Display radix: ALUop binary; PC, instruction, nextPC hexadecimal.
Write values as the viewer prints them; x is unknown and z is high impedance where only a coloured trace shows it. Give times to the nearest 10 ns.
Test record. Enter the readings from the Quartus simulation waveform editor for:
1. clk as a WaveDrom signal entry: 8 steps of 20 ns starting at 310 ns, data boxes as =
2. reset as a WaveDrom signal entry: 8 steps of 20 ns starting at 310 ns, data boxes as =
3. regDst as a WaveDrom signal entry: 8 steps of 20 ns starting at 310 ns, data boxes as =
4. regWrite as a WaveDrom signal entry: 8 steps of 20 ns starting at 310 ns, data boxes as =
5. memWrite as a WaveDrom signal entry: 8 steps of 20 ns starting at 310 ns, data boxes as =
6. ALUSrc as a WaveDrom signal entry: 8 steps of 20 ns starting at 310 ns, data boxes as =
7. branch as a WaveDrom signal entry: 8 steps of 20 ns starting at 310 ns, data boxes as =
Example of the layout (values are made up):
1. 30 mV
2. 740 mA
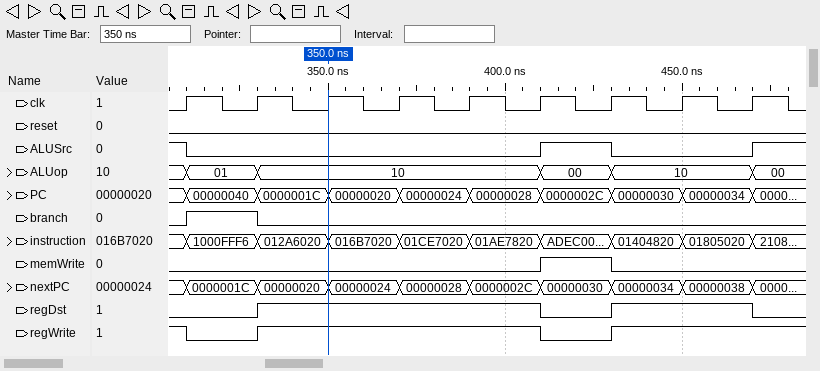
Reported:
1. {name: 'clk', wave: 'p.......'}
2. {name: 'reset', wave: '0.......'}
3. {name: 'regDst', wave: '01...01.'}
4. {name: 'regWrite', wave: '01...01.'}
5. {name: 'memWrite', wave: '0....10.'}
6. {name: 'ALUSrc', wave: '0....10.'}
7. {name: 'branch', wave: '10......'}
